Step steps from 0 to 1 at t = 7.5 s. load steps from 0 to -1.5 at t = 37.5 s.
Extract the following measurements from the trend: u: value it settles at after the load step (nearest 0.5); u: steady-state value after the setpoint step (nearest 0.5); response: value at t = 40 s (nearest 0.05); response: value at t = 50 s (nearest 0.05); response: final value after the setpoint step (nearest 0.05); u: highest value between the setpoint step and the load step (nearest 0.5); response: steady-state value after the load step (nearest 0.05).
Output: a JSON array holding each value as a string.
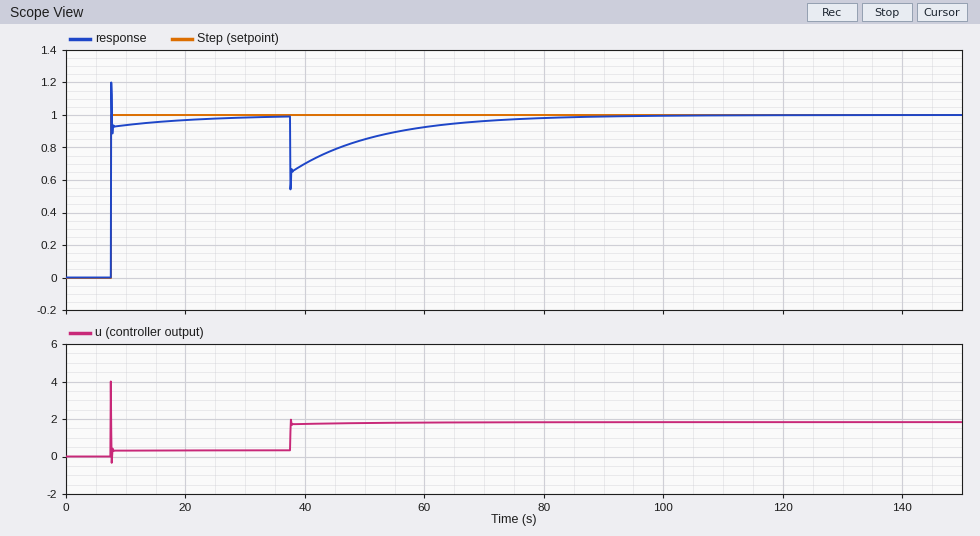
["2.0", "0.5", "0.70", "0.85", "1.00", "4.0", "1.00"]
